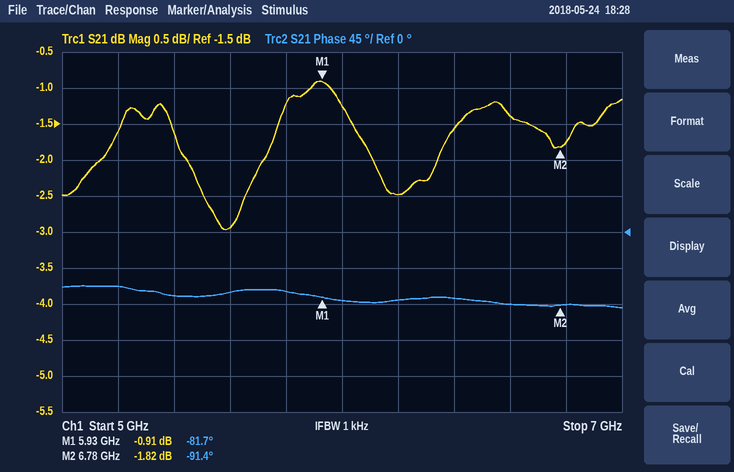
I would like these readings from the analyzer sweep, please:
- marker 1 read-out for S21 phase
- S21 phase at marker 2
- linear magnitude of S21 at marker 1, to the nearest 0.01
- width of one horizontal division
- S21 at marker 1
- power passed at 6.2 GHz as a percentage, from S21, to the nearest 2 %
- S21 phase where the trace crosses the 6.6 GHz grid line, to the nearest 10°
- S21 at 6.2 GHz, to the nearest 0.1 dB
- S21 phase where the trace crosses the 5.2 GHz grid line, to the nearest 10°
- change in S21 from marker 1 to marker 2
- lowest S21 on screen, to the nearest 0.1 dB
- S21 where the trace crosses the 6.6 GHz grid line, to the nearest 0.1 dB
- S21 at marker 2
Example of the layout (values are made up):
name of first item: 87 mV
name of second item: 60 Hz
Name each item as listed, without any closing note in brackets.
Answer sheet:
marker 1 read-out for S21 phase: -81.7°
S21 phase at marker 2: -91.4°
linear magnitude of S21 at marker 1, to the nearest 0.01: 0.90
width of one horizontal division: 200 MHz
S21 at marker 1: -0.91 dB
power passed at 6.2 GHz as a percentage, from S21, to the nearest 2 %: 56 %
S21 phase where the trace crosses the 6.6 GHz grid line, to the nearest 10°: -90°
S21 at 6.2 GHz, to the nearest 0.1 dB: -2.5 dB
S21 phase where the trace crosses the 5.2 GHz grid line, to the nearest 10°: -70°
change in S21 from marker 1 to marker 2: -0.91 dB
lowest S21 on screen, to the nearest 0.1 dB: -3.0 dB
S21 where the trace crosses the 6.6 GHz grid line, to the nearest 0.1 dB: -1.4 dB
S21 at marker 2: -1.82 dB
